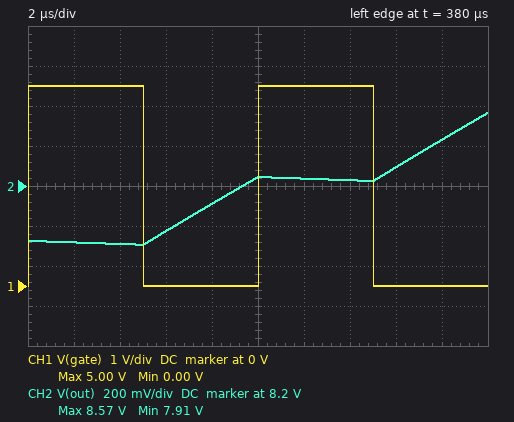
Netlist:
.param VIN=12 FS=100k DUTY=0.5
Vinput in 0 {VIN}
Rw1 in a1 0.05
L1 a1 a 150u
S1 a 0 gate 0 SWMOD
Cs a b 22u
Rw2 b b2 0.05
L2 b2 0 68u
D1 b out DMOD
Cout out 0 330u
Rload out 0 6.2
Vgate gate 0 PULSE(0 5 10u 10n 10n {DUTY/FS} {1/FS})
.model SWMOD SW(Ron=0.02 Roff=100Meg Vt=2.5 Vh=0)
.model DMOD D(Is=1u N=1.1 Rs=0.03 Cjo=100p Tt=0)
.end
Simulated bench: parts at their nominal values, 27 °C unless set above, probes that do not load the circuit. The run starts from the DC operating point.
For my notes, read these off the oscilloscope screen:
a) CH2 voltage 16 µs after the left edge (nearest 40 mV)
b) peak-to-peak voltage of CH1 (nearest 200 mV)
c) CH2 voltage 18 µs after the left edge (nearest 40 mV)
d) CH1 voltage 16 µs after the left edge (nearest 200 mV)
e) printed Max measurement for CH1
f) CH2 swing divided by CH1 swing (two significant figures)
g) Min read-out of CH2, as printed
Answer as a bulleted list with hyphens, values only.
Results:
- 8.28 V
- 5.0 V
- 8.44 V
- 0 V
- 5.00 V
- 0.13
- 7.91 V
